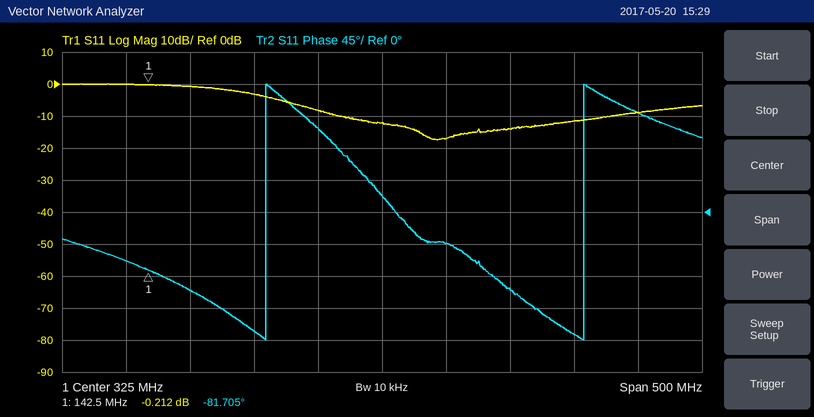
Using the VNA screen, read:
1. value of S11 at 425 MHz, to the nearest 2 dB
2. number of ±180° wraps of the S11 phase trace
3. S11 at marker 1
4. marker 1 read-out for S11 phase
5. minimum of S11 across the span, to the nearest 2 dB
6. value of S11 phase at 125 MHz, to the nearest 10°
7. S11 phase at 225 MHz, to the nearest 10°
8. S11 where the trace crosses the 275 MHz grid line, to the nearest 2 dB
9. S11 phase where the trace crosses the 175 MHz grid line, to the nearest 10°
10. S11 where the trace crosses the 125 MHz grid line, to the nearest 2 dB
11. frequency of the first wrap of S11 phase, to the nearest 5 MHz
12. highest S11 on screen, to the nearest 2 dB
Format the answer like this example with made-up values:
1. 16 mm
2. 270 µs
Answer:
1. -14 dB
2. 2
3. -0.212 dB
4. -81.705°
5. -18 dB
6. -70°
7. -170°
8. -8 dB
9. -110°
10. 0 dB
11. 235 MHz
12. 0 dB
